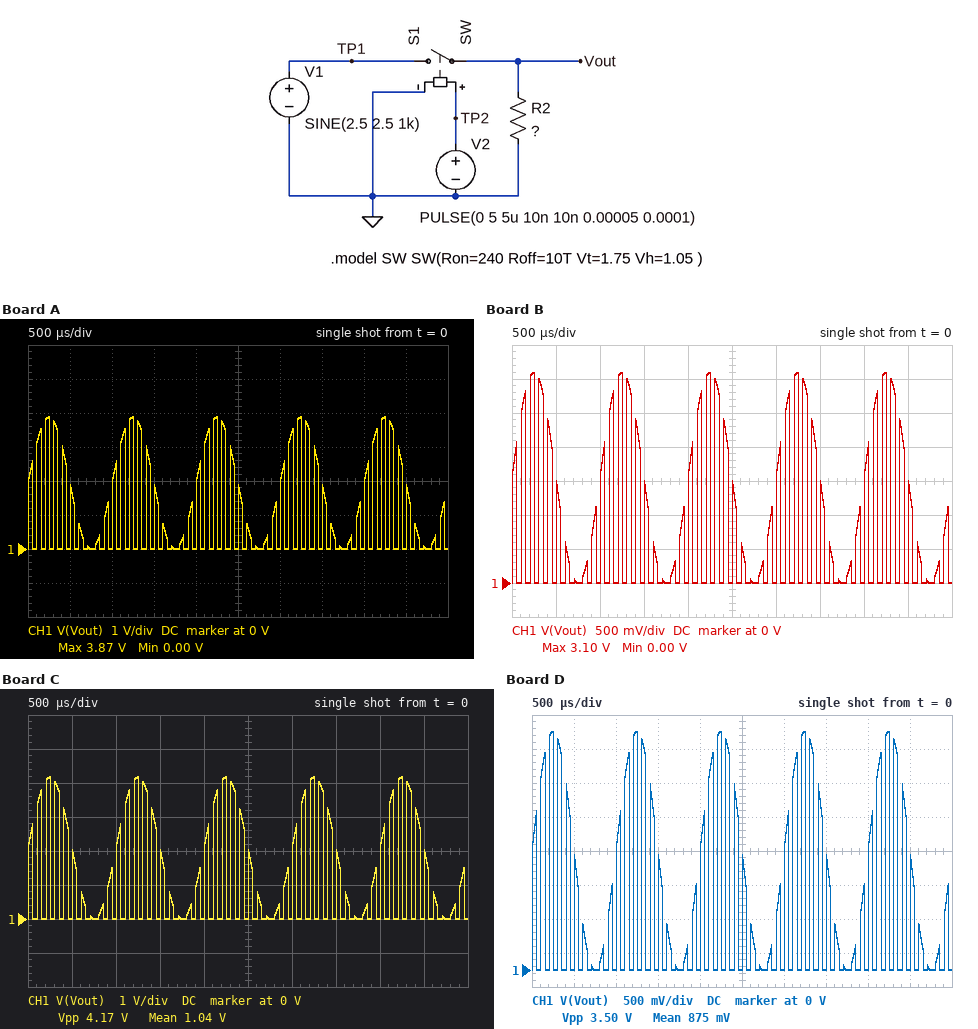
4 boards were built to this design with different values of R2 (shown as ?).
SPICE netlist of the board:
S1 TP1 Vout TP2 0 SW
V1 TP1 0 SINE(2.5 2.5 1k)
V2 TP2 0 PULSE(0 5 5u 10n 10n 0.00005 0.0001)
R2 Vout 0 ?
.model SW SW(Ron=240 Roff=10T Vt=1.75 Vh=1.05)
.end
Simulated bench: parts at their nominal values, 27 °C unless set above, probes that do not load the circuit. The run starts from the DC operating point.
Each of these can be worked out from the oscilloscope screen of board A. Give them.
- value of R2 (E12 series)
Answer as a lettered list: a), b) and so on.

a) 820 Ω
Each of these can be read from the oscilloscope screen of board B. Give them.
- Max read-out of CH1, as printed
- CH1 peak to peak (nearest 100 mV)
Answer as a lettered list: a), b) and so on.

a) 3.10 V
b) 3.1 V
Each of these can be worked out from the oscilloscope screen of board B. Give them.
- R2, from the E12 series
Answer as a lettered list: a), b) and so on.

a) 390 Ω
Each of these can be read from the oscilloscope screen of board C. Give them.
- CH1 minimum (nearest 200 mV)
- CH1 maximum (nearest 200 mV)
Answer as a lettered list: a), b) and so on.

a) 0 V
b) 4.2 V
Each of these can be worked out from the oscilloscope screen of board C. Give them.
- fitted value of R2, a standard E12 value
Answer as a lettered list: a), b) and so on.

a) 1.2 kΩ
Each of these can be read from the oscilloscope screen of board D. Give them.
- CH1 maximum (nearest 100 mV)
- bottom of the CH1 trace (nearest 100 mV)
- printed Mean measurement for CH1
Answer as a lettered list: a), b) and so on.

a) 3.5 V
b) 0 V
c) 875 mV
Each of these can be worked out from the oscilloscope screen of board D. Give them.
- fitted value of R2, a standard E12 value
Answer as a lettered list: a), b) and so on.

a) 560 Ω
